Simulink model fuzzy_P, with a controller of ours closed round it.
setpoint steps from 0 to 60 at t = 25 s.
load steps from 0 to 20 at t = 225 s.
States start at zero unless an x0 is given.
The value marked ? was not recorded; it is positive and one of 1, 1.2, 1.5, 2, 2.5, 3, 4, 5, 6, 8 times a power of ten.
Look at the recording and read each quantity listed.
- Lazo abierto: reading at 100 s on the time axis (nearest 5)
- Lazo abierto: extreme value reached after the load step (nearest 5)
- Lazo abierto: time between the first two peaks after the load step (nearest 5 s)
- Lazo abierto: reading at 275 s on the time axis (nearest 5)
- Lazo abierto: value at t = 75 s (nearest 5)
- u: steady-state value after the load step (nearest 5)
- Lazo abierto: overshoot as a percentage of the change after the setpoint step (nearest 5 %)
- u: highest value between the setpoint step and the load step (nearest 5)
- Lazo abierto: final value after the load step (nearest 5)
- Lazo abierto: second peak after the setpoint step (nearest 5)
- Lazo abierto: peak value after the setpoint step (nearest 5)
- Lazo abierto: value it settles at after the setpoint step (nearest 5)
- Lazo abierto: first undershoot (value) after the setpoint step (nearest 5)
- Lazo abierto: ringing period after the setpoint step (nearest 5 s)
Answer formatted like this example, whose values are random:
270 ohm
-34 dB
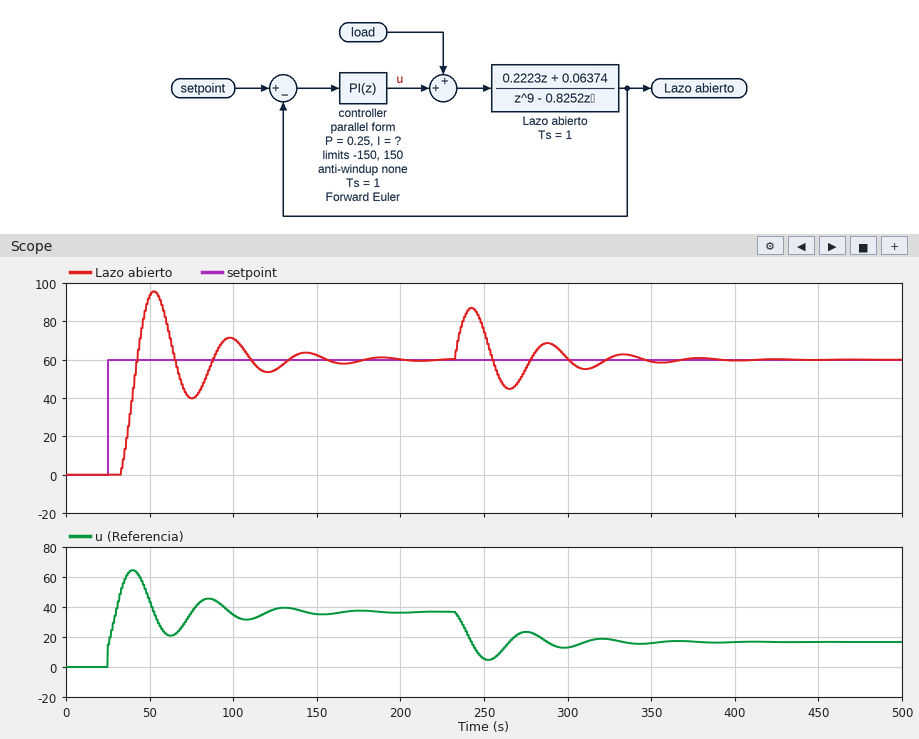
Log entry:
70
85
45 s
55
40
15
60 %
65
60
70
95
60
40
45 s
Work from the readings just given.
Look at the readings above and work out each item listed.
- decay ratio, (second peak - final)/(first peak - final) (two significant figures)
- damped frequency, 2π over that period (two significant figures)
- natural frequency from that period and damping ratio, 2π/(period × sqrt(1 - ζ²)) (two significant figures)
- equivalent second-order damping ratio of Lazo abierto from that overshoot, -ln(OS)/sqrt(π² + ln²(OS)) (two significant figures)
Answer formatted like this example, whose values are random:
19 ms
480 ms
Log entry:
0.29
0.14 rad/s
0.14 rad/s
0.16
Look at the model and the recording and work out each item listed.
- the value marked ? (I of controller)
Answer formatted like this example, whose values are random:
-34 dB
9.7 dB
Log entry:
0.08
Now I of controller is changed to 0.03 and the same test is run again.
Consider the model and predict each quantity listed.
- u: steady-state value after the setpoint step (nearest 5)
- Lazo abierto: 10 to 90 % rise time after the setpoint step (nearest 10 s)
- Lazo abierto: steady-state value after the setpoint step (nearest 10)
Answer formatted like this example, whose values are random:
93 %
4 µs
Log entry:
35
30 s
60
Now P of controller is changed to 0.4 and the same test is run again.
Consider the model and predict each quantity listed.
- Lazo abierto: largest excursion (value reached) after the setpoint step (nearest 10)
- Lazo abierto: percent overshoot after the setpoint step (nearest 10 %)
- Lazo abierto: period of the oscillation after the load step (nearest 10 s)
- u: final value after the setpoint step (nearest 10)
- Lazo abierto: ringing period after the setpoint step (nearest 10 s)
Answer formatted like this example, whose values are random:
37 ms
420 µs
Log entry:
90
50 %
40 s
40
40 s
